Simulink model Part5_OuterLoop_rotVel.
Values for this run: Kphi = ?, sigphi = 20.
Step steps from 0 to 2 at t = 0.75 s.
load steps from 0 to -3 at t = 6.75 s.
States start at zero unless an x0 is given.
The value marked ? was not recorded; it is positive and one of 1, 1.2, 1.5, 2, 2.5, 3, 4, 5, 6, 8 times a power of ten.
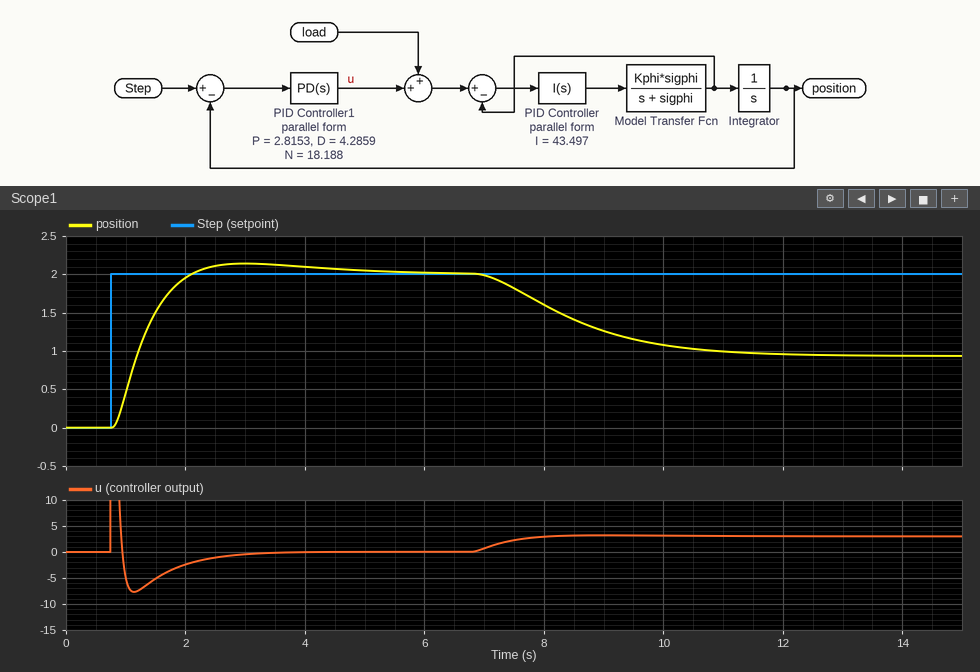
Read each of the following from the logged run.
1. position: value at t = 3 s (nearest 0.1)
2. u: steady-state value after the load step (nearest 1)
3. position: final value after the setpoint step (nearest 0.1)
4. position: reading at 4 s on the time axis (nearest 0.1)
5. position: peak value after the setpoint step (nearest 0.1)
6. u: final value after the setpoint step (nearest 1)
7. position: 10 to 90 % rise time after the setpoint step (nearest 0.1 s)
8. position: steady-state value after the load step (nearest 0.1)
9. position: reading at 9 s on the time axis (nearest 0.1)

2.1
3
2.0
2.1
2.1
0
0.9 s
0.9
1.3
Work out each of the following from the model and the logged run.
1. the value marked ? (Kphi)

0.008
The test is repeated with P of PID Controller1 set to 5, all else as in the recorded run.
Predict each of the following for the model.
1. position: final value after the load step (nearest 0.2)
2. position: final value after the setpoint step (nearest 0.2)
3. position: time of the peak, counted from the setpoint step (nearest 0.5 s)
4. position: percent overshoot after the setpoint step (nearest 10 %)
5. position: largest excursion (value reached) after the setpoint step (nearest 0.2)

1.4
2.0
1.5 s
20 %
2.4
